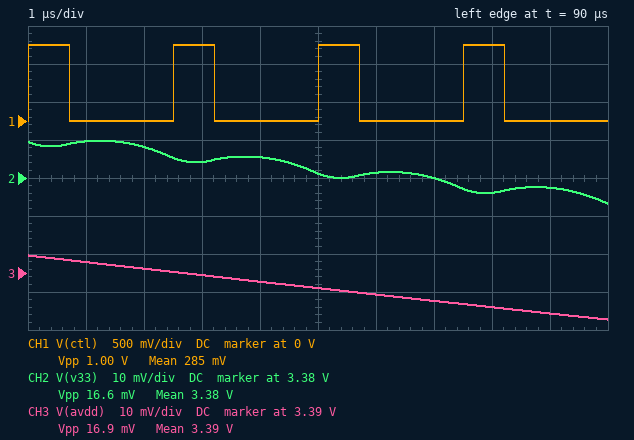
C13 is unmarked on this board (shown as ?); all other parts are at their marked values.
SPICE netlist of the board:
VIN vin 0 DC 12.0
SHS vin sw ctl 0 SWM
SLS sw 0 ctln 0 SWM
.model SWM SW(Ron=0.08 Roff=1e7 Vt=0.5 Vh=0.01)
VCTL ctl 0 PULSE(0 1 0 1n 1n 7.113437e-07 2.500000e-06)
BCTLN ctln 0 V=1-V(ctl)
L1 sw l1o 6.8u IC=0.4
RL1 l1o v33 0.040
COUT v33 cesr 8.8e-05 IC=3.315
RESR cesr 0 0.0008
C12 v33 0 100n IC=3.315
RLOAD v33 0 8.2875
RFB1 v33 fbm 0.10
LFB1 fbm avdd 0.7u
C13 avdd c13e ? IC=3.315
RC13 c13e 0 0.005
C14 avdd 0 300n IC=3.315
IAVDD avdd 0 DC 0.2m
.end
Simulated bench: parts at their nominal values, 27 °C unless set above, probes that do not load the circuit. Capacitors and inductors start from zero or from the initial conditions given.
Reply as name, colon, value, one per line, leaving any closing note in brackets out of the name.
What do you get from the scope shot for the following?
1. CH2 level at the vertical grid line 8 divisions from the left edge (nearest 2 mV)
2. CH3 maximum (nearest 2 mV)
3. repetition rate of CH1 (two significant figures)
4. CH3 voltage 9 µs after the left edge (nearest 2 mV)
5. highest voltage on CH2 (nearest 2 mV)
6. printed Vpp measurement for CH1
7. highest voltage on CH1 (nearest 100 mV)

CH2 level at the vertical grid line 8 divisions from the left edge: 3.376 V
CH3 maximum: 3.394 V
repetition rate of CH1: 400 kHz
CH3 voltage 9 µs after the left edge: 3.380 V
highest voltage on CH2: 3.390 V
printed Vpp measurement for CH1: 1.00 V
highest voltage on CH1: 1.0 V
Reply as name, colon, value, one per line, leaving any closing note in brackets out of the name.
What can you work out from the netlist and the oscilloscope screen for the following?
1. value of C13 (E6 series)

value of C13: 22 µF
